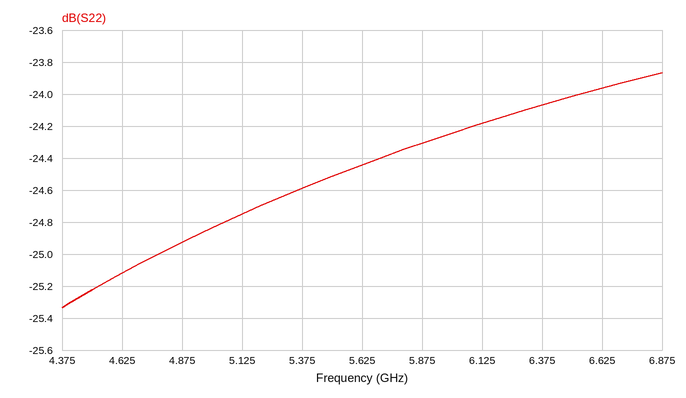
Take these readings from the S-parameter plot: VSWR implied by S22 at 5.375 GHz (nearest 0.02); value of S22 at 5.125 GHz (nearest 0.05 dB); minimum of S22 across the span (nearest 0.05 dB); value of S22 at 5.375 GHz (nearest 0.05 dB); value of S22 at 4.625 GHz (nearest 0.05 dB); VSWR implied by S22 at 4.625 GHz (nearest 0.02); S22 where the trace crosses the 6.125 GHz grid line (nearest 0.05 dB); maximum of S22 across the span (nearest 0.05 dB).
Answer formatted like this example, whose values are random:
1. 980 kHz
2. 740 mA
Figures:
1. 1.12
2. -24.75 dB
3. -25.35 dB
4. -24.60 dB
5. -25.10 dB
6. 1.12
7. -24.20 dB
8. -23.85 dB
